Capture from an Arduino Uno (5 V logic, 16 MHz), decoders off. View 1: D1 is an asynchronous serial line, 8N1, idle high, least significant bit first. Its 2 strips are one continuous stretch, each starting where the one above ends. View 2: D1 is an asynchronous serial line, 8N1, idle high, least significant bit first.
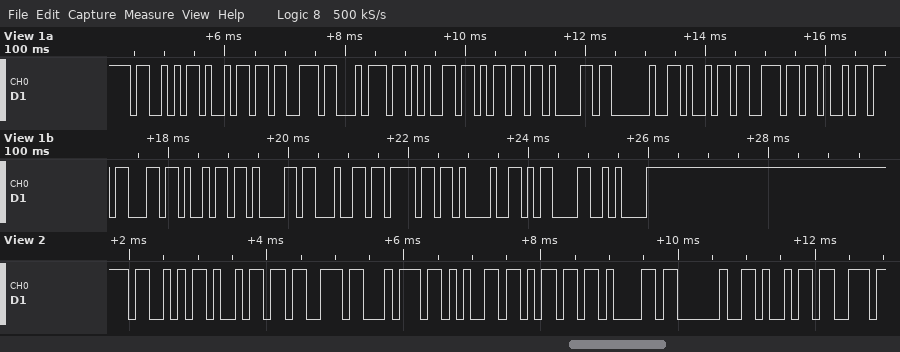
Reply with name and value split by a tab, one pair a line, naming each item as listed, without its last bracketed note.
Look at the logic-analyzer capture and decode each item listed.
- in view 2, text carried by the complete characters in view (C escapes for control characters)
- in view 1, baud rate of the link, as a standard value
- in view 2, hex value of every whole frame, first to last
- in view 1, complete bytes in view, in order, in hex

in view 2, text carried by the complete characters in view	"Sistema i"
in view 1, baud rate of the link, as a standard value	9600 baud
in view 2, hex value of every whole frame, first to last	53 69 73 74 65 6D 61 20 69
in view 1, complete bytes in view, in order, in hex	53 69 73 74 65 6D 61 20 69 6E 69 63 69 61 64 6F 21 0D 0A
